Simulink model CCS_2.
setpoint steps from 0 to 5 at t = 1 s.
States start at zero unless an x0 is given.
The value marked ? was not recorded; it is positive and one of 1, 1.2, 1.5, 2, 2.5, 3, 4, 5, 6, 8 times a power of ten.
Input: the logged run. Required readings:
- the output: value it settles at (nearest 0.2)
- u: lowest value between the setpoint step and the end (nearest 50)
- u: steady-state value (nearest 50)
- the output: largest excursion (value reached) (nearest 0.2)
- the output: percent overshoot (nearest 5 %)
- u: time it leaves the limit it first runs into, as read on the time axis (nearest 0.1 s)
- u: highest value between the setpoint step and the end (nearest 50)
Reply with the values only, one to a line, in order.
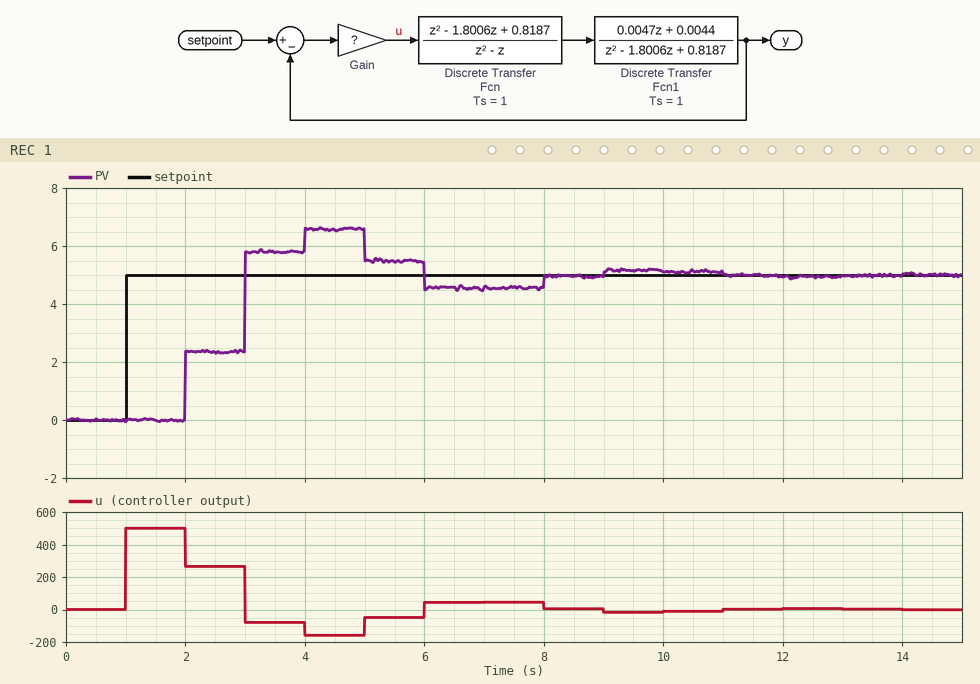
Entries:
5.0
-150
0
6.6
30 %
2.0 s
500
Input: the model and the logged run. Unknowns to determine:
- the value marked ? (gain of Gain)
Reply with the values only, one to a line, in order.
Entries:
100
